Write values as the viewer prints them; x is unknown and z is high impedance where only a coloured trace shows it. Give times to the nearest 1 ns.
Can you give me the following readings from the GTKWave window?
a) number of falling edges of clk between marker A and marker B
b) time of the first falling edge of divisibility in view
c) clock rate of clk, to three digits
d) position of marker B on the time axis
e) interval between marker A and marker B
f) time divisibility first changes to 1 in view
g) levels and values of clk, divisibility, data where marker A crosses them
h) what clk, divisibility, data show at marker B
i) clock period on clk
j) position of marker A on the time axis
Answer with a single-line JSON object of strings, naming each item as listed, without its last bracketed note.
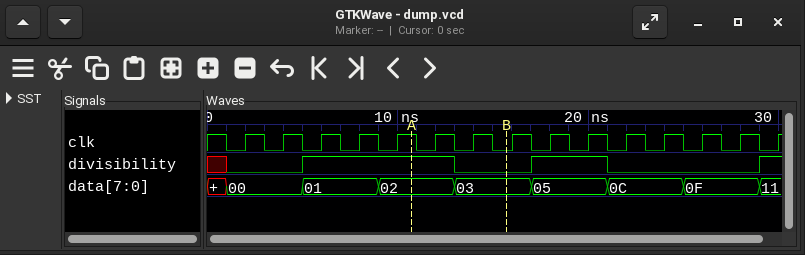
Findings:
{"number of falling edges of clk between marker A and marker B": "3", "time of the first falling edge of divisibility in view": "13 ns", "clock rate of clk, to three digits": "500 MHz", "position of marker B on the time axis": "16 ns", "interval between marker A and marker B": "5 ns", "time divisibility first changes to 1 in view": "5 ns", "levels and values of clk, divisibility, data where marker A crosses them": "clk=1, divisibility=1, data=02", "what clk, divisibility, data show at marker B": "clk=0, divisibility=0, data=03", "clock period on clk": "2 ns", "position of marker A on the time axis": "11 ns"}
